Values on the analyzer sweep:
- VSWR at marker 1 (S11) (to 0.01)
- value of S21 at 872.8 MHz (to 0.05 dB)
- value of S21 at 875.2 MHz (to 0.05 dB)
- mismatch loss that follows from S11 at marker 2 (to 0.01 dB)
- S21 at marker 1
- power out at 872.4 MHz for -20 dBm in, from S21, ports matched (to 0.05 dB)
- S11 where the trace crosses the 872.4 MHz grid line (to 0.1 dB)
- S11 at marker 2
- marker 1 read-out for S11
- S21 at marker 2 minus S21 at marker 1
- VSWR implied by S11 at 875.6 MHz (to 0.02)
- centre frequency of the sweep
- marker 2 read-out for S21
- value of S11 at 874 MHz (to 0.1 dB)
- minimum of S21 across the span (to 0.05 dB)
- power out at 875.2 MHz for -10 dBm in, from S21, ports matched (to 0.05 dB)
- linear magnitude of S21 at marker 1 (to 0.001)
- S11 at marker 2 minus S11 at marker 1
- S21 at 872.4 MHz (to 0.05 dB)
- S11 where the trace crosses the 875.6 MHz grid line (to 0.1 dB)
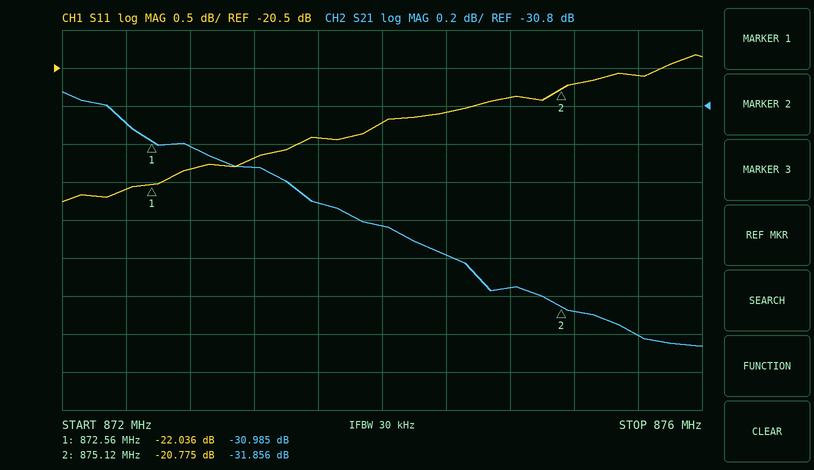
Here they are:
1.17
-31.00 dB
-31.90 dB
0.04 dB
-30.985 dB
-50.90 dBm
-22.1 dB
-20.775 dB
-22.036 dB
-0.871 dB
1.20
874 MHz
-31.856 dB
-21.2 dB
-32.05 dB
-41.90 dBm
0.028
1.261 dB
-30.90 dB
-20.6 dB
